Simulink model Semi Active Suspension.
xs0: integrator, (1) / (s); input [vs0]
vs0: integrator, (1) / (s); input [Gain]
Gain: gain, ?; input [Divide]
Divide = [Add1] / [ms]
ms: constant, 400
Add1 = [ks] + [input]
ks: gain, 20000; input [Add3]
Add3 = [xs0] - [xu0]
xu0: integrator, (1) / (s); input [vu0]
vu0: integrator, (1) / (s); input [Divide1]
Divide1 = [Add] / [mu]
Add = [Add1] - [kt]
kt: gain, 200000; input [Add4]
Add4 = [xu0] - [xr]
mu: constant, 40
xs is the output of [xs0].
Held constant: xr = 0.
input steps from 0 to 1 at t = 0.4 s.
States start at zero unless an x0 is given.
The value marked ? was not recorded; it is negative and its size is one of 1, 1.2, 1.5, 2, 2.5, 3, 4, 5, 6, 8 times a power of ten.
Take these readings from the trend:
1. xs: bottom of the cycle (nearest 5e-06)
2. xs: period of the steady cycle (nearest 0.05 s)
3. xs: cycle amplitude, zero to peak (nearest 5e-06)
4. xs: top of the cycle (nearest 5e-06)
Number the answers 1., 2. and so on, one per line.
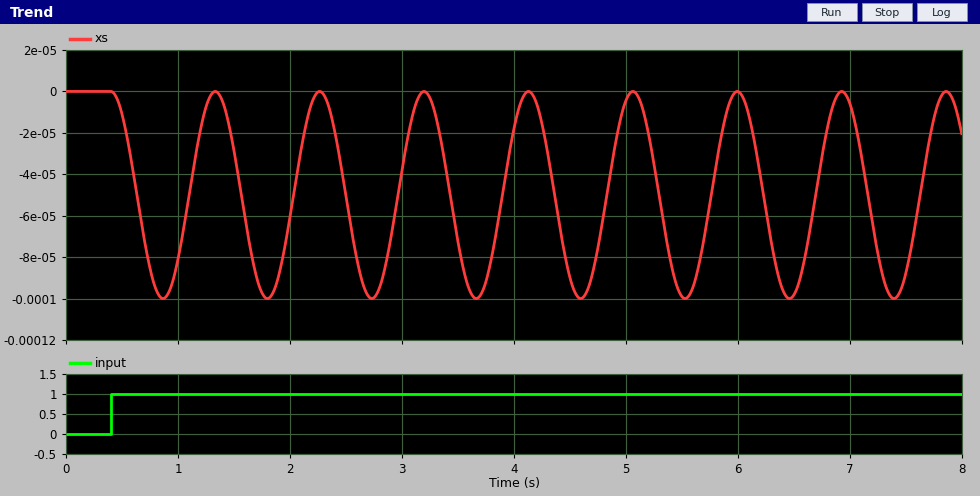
1. -0.000100
2. 0.95 s
3. 0.000050
4. 0.000000
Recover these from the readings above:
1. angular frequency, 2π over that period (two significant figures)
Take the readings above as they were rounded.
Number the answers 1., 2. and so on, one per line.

1. 6.6 rad/s
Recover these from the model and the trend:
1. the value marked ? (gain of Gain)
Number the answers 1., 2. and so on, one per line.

1. -1
